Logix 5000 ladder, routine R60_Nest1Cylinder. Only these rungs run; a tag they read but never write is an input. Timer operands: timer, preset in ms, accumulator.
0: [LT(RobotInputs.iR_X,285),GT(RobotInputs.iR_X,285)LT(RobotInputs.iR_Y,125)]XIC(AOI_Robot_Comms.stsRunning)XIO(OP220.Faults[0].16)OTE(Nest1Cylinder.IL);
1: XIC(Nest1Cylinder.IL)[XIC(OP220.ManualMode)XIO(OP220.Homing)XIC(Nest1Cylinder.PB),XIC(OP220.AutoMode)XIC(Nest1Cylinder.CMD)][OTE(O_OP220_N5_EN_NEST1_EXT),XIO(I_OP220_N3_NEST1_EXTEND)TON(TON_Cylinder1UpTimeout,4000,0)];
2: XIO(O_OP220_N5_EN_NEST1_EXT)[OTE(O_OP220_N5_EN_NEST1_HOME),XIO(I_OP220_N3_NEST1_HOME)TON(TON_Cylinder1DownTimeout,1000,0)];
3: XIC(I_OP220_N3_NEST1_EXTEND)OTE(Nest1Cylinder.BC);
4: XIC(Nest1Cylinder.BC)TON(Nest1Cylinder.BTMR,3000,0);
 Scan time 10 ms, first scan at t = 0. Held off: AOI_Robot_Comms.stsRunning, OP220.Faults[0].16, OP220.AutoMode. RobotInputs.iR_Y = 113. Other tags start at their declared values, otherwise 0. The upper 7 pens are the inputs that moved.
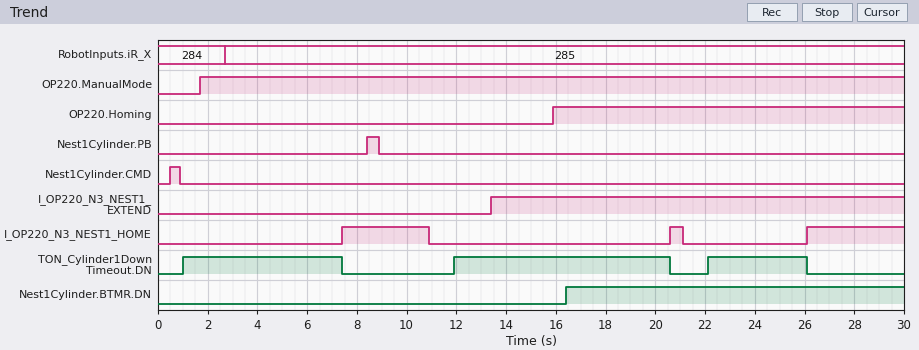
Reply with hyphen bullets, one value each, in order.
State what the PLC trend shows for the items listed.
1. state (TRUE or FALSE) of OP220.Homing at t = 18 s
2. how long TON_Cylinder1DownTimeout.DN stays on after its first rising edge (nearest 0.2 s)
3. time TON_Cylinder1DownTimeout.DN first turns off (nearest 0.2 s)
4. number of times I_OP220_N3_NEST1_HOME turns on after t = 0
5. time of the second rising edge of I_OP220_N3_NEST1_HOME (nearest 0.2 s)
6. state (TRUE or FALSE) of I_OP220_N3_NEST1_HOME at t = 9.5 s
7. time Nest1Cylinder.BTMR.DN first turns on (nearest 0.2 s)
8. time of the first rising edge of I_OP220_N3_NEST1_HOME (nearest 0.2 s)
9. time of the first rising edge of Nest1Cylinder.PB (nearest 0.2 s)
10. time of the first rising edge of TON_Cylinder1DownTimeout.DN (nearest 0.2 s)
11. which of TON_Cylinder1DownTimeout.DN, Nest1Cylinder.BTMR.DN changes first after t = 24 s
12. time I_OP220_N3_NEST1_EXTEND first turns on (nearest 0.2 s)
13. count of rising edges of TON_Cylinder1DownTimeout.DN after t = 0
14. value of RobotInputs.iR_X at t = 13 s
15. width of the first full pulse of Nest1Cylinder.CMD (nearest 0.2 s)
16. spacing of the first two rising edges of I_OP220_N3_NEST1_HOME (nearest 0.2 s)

- TRUE
- 6.4 s
- 7.4 s
- 3
- 20.6 s
- TRUE
- 16.4 s
- 7.4 s
- 8.4 s
- 1.0 s
- TON_Cylinder1DownTimeout.DN
- 13.4 s
- 3
- 285
- 0.4 s
- 13.2 s
